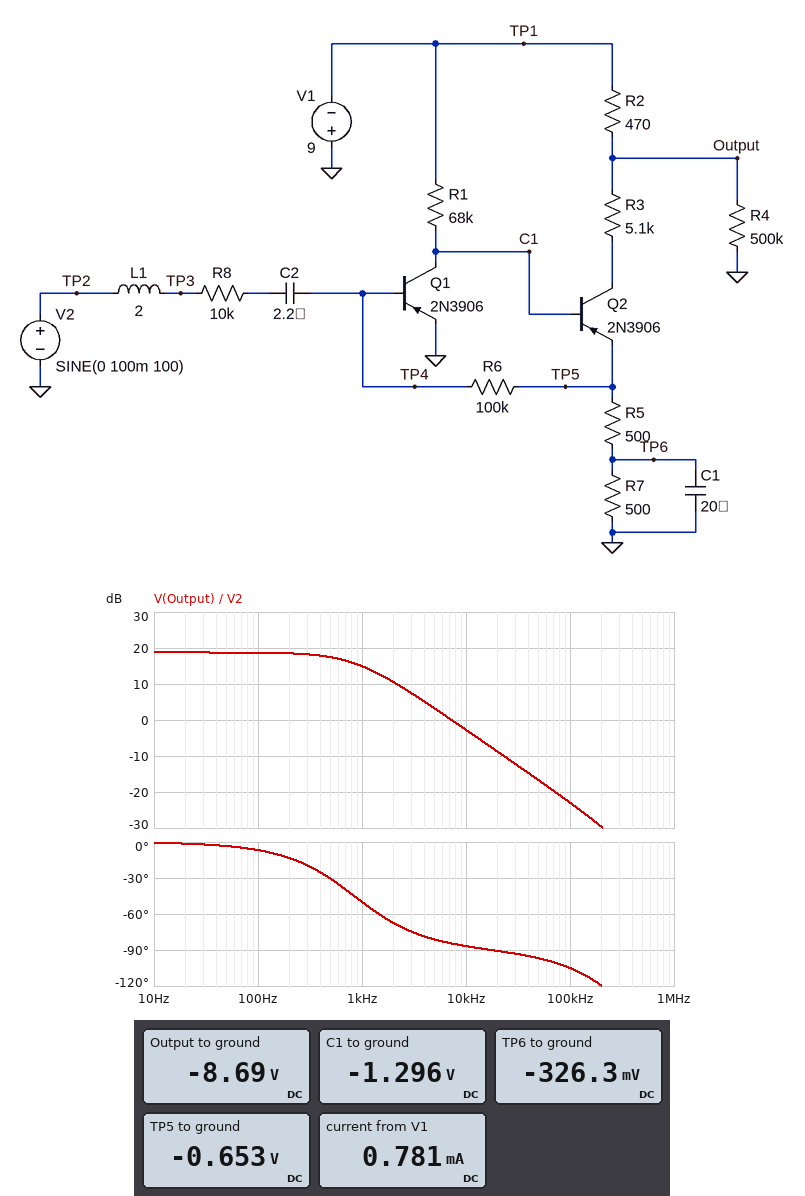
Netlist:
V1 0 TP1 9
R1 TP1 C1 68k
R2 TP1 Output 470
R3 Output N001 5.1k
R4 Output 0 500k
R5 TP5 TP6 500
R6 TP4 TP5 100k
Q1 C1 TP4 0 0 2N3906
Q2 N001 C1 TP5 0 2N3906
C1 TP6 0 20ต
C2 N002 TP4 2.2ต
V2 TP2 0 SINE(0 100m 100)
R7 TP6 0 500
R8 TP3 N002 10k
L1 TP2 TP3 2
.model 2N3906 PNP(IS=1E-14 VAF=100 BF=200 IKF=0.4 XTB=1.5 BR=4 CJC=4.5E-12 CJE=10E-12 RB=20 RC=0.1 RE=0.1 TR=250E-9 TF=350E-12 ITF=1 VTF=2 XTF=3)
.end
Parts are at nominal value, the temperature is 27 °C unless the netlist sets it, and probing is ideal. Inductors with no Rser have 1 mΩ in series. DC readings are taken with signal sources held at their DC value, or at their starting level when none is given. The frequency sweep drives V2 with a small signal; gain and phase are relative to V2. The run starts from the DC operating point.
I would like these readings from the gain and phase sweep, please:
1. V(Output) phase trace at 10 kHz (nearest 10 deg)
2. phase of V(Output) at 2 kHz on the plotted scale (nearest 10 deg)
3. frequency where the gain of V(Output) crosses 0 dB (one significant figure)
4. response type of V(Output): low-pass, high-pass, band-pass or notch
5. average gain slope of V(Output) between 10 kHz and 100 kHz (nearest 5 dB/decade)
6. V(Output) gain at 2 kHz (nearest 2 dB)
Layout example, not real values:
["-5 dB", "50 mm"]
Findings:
["-90 deg", "-70 deg", "7 kHz", "low-pass", "-20 dB/decade", "10 dB"]
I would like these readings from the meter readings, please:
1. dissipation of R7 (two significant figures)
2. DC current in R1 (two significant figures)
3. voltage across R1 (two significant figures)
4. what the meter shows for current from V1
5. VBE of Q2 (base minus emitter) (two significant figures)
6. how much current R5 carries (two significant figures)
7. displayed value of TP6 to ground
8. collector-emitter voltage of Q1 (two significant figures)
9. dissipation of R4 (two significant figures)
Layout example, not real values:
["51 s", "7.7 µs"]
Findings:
["210 µW", "110 µA", "7.7 V", "0.781 mA", "-640 mV", "650 µA", "-326.3 mV", "-1.3 V", "150 µW"]
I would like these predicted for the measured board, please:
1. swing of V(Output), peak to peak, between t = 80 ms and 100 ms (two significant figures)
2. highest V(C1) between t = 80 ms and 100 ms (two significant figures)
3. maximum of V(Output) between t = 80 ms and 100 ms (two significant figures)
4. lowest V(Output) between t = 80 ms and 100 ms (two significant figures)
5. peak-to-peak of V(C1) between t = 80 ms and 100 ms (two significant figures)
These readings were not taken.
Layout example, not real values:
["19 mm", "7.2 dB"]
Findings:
["660 mV", "-52 mV", "-8.3 V", "-9.0 V", "1.7 V"]
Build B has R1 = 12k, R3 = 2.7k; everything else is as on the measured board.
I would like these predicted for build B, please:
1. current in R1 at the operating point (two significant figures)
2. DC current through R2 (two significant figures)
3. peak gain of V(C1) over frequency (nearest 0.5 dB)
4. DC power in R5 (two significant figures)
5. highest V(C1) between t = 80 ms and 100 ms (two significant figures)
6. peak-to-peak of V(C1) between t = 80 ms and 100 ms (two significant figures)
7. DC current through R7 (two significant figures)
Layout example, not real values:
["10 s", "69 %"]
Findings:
["620 µA", "960 µA", "19.5 dB", "450 µW", "-100 mV", "2.3 V", "950 µA"]
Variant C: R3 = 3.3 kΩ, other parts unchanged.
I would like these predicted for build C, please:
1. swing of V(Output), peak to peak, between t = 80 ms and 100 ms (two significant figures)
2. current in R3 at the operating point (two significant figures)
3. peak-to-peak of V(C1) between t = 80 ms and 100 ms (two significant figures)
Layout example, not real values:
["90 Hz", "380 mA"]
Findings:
["940 mV", "650 µA", "2.0 V"]
